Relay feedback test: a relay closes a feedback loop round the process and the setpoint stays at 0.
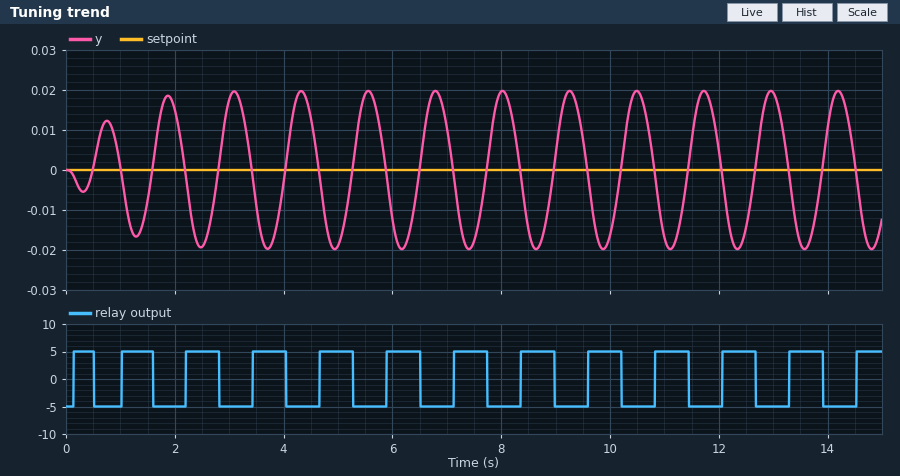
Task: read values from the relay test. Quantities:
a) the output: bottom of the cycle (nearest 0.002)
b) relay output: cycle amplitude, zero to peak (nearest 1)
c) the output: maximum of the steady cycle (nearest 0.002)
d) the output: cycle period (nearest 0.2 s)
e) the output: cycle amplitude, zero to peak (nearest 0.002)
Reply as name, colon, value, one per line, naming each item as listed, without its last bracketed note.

the output: bottom of the cycle: -0.020
relay output: cycle amplitude, zero to peak: 5
the output: maximum of the steady cycle: 0.020
the output: cycle period: 1.2 s
the output: cycle amplitude, zero to peak: 0.020
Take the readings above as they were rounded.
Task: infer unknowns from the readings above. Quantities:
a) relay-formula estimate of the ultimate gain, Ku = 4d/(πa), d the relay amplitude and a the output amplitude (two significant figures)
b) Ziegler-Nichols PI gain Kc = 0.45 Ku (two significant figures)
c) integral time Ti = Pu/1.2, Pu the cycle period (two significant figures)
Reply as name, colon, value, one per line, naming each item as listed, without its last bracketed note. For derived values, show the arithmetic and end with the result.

relay-formula estimate of the ultimate gain, Ku = 4d/(πa), d the relay amplitude and a the output amplitude: 4 × 5 / (π × 0.02) = 320
Ziegler-Nichols PI gain Kc = 0.45 Ku: 0.45 × 320 = 140
integral time Ti = Pu/1.2, Pu the cycle period: 1.2 / 1.2 = 1.0 s
